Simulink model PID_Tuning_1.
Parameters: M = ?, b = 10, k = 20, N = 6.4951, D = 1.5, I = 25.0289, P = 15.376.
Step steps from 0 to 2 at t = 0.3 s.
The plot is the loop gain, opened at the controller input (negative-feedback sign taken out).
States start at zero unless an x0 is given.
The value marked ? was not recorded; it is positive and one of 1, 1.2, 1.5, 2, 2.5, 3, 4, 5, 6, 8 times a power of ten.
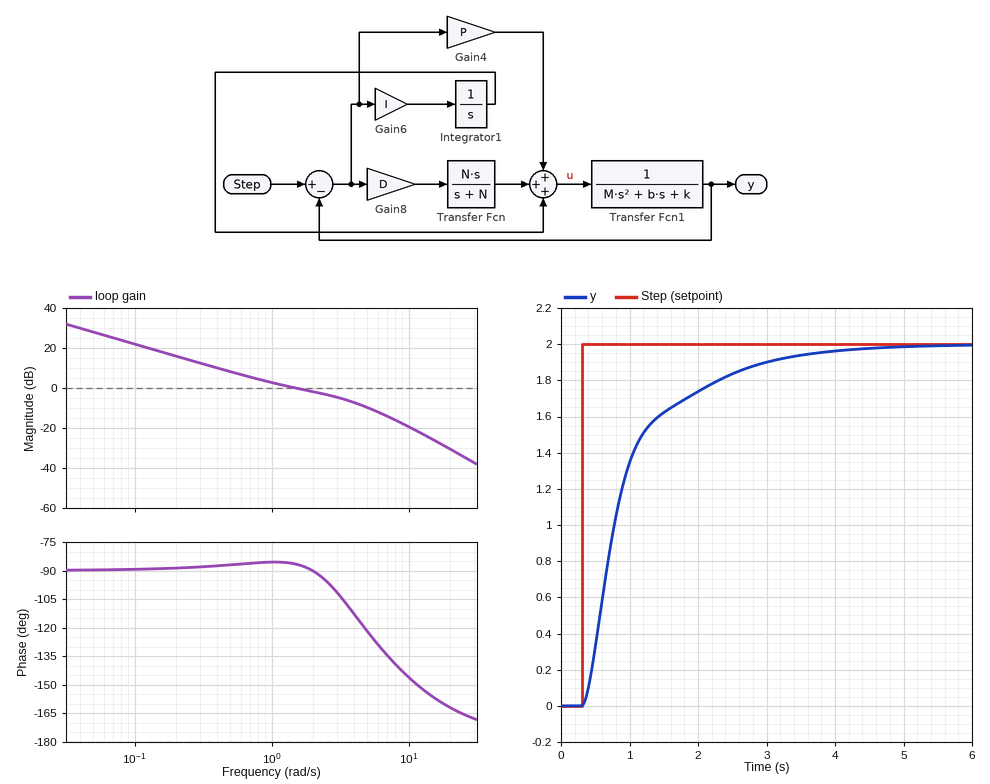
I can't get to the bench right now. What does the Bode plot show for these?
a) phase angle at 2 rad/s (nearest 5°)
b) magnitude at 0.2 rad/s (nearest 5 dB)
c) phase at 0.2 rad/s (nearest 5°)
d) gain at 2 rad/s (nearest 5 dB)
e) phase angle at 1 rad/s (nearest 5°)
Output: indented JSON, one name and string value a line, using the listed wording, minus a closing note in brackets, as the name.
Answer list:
{
  "phase angle at 2 rad/s": "-90°",
  "magnitude at 0.2 rad/s": "15 dB",
  "phase at 0.2 rad/s": "-90°",
  "gain at 2 rad/s": "0 dB",
  "phase angle at 1 rad/s": "-85°"
}
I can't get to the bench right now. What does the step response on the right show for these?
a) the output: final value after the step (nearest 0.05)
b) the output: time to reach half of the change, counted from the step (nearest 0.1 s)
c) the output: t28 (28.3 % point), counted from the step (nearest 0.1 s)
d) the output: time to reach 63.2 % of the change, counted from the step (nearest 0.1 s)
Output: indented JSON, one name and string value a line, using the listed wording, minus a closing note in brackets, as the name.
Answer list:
{
  "the output: final value after the step": "2.00",
  "the output: time to reach half of the change, counted from the step": "0.5 s",
  "the output: t28 (28.3 % point), counted from the step": "0.3 s",
  "the output: time to reach 63.2 % of the change, counted from the step": "0.6 s"
}
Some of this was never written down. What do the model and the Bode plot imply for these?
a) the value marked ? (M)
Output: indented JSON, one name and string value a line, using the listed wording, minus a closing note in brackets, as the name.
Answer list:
{
  "the value marked ?": "2"
}
